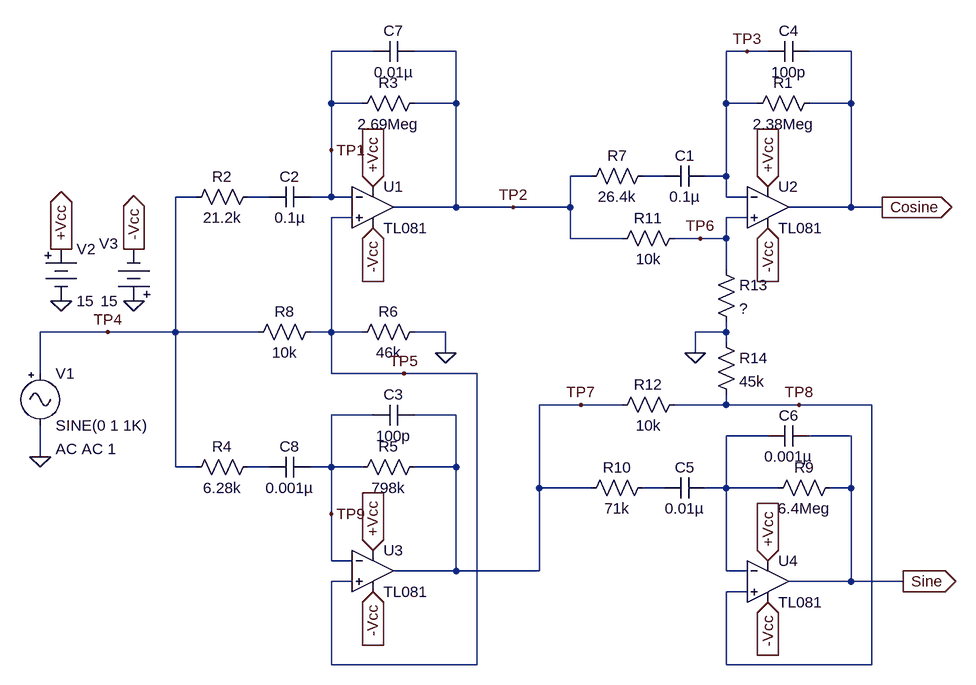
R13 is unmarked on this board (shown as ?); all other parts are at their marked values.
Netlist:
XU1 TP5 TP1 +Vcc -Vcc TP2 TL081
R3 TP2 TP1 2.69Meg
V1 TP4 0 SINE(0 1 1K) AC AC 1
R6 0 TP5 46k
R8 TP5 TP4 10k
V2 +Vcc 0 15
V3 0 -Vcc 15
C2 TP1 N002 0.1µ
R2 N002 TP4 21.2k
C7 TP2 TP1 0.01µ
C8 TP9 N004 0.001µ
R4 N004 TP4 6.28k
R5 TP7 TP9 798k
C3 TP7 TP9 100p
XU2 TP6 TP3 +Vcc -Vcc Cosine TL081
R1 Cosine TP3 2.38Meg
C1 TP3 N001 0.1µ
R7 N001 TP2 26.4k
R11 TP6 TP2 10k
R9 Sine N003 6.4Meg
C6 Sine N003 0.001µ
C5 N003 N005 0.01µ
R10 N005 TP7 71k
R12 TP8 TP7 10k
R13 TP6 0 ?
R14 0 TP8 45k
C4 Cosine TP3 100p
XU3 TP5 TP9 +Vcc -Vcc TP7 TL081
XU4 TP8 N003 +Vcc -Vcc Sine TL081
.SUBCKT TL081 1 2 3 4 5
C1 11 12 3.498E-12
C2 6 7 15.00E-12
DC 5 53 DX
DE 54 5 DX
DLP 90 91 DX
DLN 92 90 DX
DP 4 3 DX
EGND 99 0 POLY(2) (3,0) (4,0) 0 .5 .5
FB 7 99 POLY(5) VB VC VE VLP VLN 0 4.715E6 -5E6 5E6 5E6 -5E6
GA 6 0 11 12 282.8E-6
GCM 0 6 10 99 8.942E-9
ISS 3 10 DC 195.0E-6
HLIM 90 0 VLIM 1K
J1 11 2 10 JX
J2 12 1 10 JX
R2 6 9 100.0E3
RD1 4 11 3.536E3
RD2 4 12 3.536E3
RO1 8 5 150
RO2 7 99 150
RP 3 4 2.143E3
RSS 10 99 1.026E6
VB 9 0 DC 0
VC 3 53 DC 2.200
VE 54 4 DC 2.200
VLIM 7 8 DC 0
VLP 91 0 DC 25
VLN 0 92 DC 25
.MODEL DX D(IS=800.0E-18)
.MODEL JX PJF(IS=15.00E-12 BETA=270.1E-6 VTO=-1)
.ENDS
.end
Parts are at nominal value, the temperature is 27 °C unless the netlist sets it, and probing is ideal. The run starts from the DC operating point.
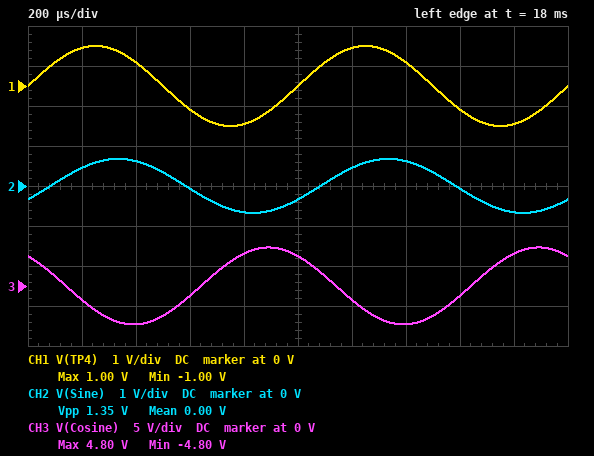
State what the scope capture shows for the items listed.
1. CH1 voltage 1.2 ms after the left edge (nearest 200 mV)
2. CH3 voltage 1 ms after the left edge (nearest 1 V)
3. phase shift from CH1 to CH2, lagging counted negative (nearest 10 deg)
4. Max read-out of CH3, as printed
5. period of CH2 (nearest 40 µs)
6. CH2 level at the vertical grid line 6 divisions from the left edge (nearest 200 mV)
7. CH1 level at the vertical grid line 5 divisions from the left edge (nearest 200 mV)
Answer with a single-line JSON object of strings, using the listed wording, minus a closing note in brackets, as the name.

{"CH1 voltage 1.2 ms after the left edge": "1.0 V", "CH3 voltage 1 ms after the left edge": "4 V", "phase shift from CH1 to CH2, lagging counted negative": "-30 deg", "Max read-out of CH3, as printed": "4.80 V", "period of CH2": "1.00 ms", "CH2 level at the vertical grid line 6 divisions from the left edge": "400 mV", "CH1 level at the vertical grid line 5 divisions from the left edge": "0 V"}
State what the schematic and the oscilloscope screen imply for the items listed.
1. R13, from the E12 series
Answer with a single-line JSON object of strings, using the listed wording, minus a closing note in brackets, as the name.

{"R13, from the E12 series": "68 kΩ"}
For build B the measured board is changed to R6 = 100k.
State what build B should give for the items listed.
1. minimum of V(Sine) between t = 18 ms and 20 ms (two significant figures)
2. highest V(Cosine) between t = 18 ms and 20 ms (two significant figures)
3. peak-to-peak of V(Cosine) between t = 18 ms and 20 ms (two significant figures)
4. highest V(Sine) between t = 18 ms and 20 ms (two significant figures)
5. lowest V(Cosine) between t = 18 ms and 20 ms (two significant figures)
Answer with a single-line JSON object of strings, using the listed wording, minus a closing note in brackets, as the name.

{"minimum of V(Sine) between t = 18 ms and 20 ms": "-650 mV", "highest V(Cosine) between t = 18 ms and 20 ms": "5.3 V", "peak-to-peak of V(Cosine) between t = 18 ms and 20 ms": "11 V", "highest V(Sine) between t = 18 ms and 20 ms": "660 mV", "lowest V(Cosine) between t = 18 ms and 20 ms": "-5.3 V"}
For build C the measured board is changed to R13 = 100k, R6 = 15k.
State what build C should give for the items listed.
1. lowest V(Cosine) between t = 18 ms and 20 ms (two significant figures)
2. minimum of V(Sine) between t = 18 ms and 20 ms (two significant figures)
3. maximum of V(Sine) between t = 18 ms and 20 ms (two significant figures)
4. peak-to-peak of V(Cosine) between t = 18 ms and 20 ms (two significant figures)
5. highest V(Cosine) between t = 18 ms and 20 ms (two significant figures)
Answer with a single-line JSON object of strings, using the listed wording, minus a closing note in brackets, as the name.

{"lowest V(Cosine) between t = 18 ms and 20 ms": "-2.6 V", "minimum of V(Sine) between t = 18 ms and 20 ms": "-1.3 V", "maximum of V(Sine) between t = 18 ms and 20 ms": "1.3 V", "peak-to-peak of V(Cosine) between t = 18 ms and 20 ms": "5.2 V", "highest V(Cosine) between t = 18 ms and 20 ms": "2.6 V"}
